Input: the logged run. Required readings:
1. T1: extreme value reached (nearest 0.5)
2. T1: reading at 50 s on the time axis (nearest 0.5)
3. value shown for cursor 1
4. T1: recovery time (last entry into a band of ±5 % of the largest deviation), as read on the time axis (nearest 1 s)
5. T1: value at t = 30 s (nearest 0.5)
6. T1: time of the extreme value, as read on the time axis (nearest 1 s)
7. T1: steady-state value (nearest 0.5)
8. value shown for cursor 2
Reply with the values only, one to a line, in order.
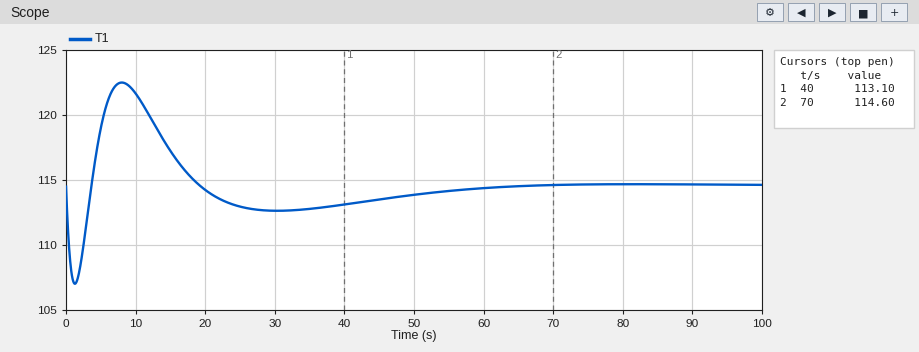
122.5
114.0
113.10
56 s
112.5
8 s
114.5
114.60
